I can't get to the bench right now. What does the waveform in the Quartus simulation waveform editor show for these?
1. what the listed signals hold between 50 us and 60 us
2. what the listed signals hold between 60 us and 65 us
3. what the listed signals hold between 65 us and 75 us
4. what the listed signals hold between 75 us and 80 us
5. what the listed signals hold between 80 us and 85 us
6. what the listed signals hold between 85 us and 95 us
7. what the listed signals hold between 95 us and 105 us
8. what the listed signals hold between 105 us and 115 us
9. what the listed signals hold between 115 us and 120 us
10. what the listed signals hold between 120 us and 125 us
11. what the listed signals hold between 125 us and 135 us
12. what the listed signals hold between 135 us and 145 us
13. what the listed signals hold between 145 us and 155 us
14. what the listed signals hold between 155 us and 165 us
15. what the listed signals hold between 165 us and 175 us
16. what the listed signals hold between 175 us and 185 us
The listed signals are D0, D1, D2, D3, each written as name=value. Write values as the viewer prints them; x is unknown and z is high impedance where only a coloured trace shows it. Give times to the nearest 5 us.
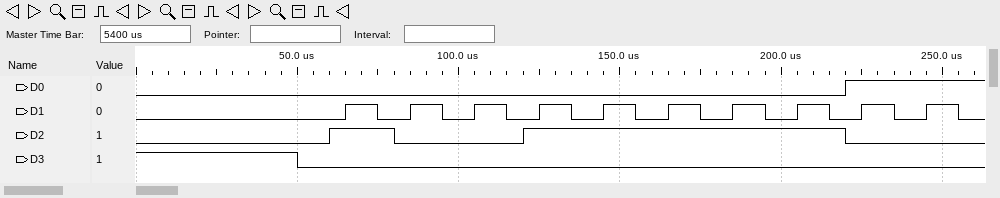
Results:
D0=0, D1=0, D2=0, D3=0
D0=0, D1=0, D2=1, D3=0
D0=0, D1=1, D2=1, D3=0
D0=0, D1=0, D2=1, D3=0
D0=0, D1=0, D2=0, D3=0
D0=0, D1=1, D2=0, D3=0
D0=0, D1=0, D2=0, D3=0
D0=0, D1=1, D2=0, D3=0
D0=0, D1=0, D2=0, D3=0
D0=0, D1=0, D2=1, D3=0
D0=0, D1=1, D2=1, D3=0
D0=0, D1=0, D2=1, D3=0
D0=0, D1=1, D2=1, D3=0
D0=0, D1=0, D2=1, D3=0
D0=0, D1=1, D2=1, D3=0
D0=0, D1=0, D2=1, D3=0
